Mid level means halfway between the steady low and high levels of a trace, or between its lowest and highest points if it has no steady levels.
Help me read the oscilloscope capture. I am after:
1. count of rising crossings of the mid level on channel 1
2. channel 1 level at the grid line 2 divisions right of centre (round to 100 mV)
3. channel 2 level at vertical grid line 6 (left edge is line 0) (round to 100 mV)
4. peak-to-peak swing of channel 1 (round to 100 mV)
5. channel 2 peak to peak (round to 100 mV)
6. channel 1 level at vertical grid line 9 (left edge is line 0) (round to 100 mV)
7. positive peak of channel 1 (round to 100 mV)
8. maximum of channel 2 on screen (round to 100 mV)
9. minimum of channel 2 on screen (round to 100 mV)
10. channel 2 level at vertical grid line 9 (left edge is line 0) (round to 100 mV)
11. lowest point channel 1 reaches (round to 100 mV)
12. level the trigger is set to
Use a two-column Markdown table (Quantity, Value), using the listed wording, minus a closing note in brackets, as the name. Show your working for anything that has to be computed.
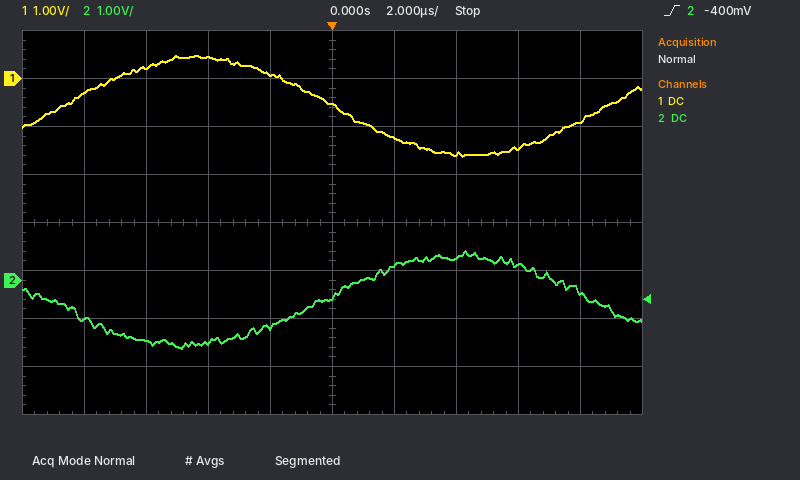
| Quantity | Value |
|---|---|
| count of rising crossings of the mid level on channel 1 | 2 |
| channel 1 level at the grid line 2 divisions right of centre | -1.6 V |
| channel 2 level at vertical grid line 6 (left edge is line 0) | 300 mV |
| peak-to-peak swing of channel 1 | 500 mV − (-1.6 V) = 2.1 V |
| channel 2 peak to peak | 600 mV − (-1.4 V) = 2.0 V |
| channel 1 level at vertical grid line 9 (left edge is line 0) | -900 mV |
| positive peak of channel 1 | 500 mV |
| maximum of channel 2 on screen | 600 mV |
| minimum of channel 2 on screen | -1.4 V |
| channel 2 level at vertical grid line 9 (left edge is line 0) | -200 mV |
| lowest point channel 1 reaches | -1.6 V |
| level the trigger is set to | -400 mV |
